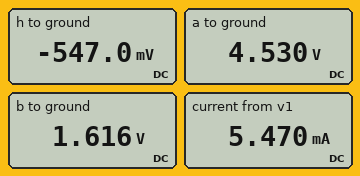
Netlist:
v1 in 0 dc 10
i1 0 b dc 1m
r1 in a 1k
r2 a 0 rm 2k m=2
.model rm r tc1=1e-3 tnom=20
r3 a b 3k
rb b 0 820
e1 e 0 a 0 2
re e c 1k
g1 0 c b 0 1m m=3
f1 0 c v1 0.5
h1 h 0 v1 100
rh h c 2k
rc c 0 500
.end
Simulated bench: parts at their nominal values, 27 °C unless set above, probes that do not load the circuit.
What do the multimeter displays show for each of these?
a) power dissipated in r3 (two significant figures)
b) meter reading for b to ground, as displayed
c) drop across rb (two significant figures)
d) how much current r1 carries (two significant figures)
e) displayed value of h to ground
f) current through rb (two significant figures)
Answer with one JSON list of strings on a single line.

["2.8 mW", "1.616 V", "1.6 V", "5.5 mA", "-547.0 mV", "2.0 mA"]
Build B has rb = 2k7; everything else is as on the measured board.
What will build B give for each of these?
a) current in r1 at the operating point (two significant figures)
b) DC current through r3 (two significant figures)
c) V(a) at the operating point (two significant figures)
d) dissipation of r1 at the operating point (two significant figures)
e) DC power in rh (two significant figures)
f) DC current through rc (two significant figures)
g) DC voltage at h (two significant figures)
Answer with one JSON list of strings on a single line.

["5.2 mA", "370 µA", "4.8 V", "27 mW", "16 mW", "10 mA", "-520 mV"]
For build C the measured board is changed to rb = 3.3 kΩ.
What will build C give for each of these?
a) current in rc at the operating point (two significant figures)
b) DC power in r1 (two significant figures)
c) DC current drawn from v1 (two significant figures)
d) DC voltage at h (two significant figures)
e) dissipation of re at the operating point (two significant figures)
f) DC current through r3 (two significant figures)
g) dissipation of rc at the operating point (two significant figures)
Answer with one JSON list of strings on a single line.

["11 mA", "26 mW", "5.1 mA", "-510 mV", "18 mW", "250 µA", "61 mW"]
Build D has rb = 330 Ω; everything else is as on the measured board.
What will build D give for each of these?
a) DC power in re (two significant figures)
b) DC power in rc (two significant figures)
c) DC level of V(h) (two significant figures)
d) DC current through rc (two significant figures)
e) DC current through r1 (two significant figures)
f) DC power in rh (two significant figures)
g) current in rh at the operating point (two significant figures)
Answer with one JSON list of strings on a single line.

["43 mW", "10 mW", "-560 mV", "4.5 mA", "5.6 mA", "4.0 mW", "1.4 mA"]
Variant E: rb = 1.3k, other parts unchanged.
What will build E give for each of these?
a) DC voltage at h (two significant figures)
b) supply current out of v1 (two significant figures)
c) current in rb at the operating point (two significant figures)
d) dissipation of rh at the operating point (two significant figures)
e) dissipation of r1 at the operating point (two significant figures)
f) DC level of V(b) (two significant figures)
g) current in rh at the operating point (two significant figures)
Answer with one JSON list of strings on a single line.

["-540 mV", "5.4 mA", "1.8 mA", "9.3 mW", "29 mW", "2.3 V", "2.2 mA"]
